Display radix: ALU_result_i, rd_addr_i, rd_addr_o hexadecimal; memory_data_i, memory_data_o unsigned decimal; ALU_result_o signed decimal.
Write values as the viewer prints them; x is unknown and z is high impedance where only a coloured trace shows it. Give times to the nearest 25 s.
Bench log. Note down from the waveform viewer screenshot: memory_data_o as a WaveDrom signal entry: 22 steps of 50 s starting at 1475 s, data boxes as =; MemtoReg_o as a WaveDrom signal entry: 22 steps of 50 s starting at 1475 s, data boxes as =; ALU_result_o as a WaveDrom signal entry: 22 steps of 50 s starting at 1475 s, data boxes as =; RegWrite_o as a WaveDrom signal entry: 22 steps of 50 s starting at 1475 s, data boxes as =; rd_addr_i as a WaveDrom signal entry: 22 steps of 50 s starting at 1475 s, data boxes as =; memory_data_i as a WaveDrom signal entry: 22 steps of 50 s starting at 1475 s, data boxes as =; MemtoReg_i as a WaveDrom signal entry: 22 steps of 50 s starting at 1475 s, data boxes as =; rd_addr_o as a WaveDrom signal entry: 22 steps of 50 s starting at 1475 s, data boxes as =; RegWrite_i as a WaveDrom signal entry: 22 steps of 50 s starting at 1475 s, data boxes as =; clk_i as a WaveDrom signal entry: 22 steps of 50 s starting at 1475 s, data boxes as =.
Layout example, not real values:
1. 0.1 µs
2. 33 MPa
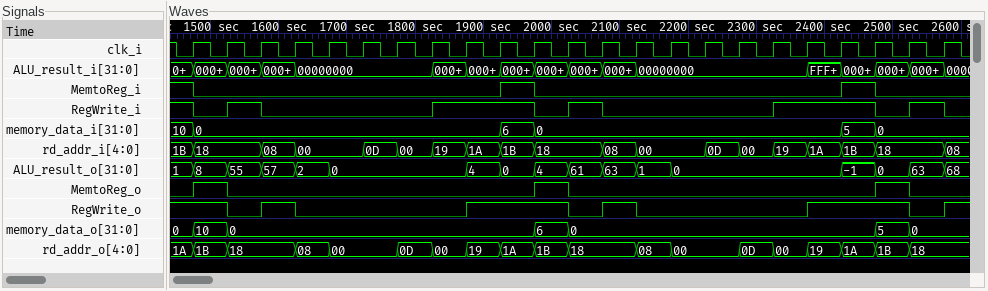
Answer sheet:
1. {name: 'memory_data_o', wave: '==........==........==', data: '10 0 6 0 5 0'}
2. {name: 'MemtoReg_o', wave: '10........10........10'}
3. {name: 'ALU_result_o', wave: '=====...=======....===', data: '8 55 57 2 0 4 0 4 61 63 1 0 -1 0 63'}
4. {name: 'RegWrite_o', wave: '1010....1..010....1..0'}
5. {name: 'rd_addr_i', wave: '=.==.======.==.======.', data: '18 08 00 0D 00 19 1A 1B 18 08 00 0D 00 19 1A 1B 18'}
6. {name: 'memory_data_i', wave: '=........==........==.', data: '0 6 0 5 0'}
7. {name: 'MemtoReg_i', wave: '0........10........10.'}
8. {name: 'rd_addr_o', wave: '==.==.======.==.======', data: '1B 18 08 00 0D 00 19 1A 1B 18 08 00 0D 00 19 1A 1B 18'}
9. {name: 'RegWrite_i', wave: '010....1..010....1..01'}
10. {name: 'clk_i', wave: 'p.....................'}
